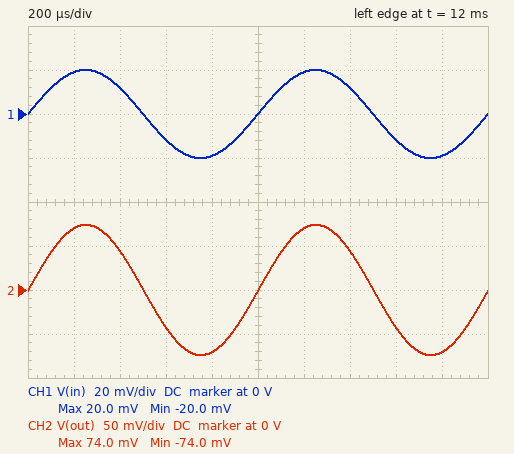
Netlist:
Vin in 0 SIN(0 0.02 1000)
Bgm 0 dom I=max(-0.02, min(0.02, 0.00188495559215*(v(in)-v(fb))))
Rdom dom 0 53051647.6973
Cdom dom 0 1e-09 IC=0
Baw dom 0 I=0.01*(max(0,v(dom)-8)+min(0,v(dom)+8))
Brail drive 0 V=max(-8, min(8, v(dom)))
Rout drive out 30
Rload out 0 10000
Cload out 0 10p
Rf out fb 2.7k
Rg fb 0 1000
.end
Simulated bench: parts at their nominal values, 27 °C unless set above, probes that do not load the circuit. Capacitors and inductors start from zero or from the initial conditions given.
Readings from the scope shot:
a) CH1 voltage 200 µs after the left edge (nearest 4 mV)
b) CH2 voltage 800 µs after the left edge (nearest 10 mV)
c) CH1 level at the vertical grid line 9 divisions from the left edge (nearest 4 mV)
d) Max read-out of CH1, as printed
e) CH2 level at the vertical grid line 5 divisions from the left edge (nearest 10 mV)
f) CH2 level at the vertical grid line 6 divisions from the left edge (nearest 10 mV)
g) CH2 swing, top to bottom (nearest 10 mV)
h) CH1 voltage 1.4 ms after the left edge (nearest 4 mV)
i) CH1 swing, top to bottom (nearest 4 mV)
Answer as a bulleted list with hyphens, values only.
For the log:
- 20 mV
- -70 mV
- -20 mV
- 20.0 mV
- 0 V
- 70 mV
- 150 mV
- 12 mV
- 40 mV
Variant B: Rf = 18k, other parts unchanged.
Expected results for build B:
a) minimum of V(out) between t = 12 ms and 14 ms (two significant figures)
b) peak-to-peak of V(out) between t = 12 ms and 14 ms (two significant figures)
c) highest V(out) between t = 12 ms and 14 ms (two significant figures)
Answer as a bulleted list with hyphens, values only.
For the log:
- -380 mV
- 760 mV
- 380 mV
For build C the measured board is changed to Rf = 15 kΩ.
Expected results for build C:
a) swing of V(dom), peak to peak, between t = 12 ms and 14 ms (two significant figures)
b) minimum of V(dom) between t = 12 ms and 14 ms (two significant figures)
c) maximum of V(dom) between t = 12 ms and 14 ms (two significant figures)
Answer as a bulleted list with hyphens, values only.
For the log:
- 640 mV
- -320 mV
- 320 mV
